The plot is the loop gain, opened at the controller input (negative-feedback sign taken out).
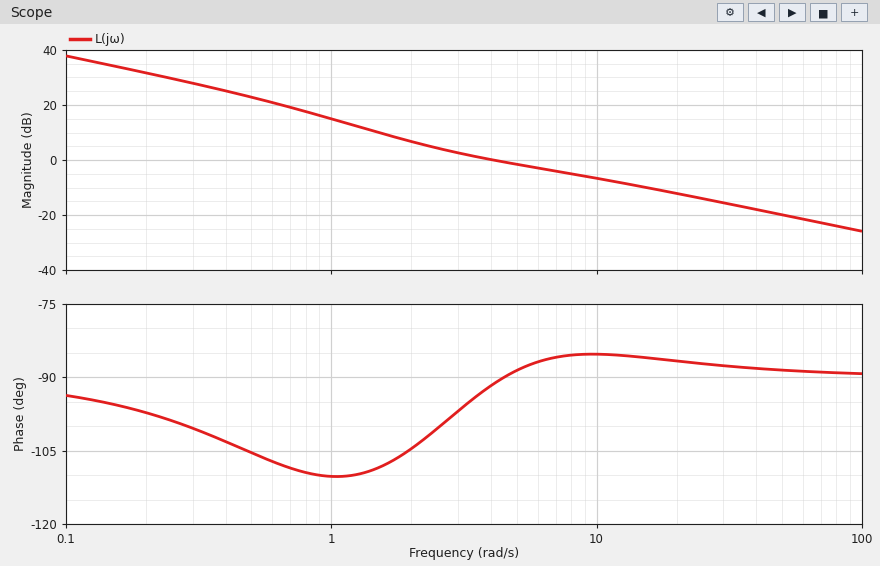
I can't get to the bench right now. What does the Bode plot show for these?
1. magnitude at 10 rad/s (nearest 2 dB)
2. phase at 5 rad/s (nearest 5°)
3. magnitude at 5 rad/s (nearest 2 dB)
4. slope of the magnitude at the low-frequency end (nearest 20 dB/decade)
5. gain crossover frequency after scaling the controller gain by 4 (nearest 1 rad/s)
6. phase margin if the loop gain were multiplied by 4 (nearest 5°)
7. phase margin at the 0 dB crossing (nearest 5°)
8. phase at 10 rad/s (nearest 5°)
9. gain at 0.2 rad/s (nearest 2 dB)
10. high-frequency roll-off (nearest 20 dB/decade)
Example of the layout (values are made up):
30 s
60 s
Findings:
-6 dB
-90°
-2 dB
-20 dB/decade
20 rad/s
95°
90°
-85°
32 dB
-20 dB/decade
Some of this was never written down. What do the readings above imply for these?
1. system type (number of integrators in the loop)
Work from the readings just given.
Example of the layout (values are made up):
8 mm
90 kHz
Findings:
1
